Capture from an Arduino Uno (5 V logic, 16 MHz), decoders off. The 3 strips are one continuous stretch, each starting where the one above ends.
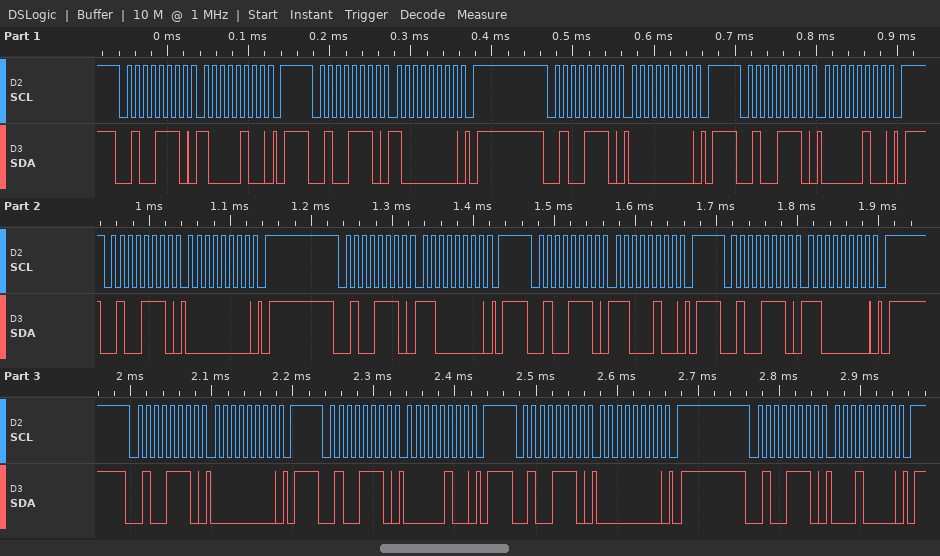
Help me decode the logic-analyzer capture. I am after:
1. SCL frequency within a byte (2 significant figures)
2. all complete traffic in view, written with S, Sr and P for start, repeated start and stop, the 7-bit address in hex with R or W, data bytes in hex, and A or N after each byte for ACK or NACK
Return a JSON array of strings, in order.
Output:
["100 kHz", "S 27W A 84 A P S 27W A 80 A P S 27W A 00 A P S 27W A 04 A P S 27W A 00 A P S 27W A C0 A P S 27W A C4 A P S 27W A C0 A P S 27W A 00 A P S 27W A 04 A P S 27W A 00 A P S 27W A 10 A P"]
